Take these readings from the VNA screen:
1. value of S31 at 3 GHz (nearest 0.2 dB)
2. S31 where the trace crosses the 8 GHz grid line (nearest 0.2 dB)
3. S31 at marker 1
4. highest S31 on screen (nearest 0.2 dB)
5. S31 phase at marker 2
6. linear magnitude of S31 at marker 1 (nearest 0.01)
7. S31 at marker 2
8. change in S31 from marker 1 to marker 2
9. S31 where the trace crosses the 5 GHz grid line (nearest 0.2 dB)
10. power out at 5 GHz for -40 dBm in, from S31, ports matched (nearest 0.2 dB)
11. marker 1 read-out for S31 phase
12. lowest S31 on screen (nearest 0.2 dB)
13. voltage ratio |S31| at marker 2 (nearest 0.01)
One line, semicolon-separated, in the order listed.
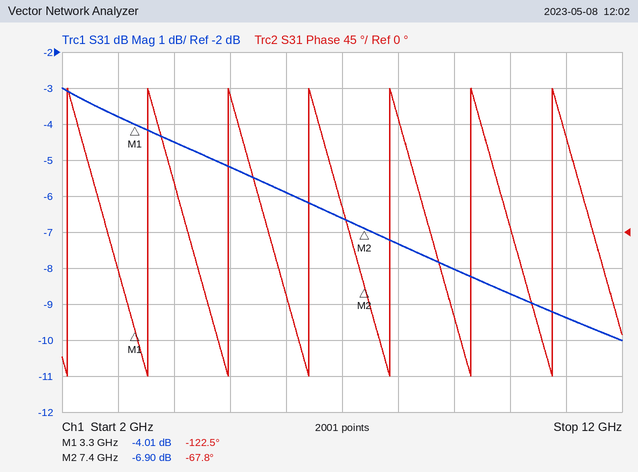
-3.8 dB; -7.4 dB; -4.01 dB; -3.0 dB; -67.8°; 0.63; -6.90 dB; -2.89 dB; -5.2 dB; -45.2 dBm; -122.5°; -10.0 dB; 0.45
